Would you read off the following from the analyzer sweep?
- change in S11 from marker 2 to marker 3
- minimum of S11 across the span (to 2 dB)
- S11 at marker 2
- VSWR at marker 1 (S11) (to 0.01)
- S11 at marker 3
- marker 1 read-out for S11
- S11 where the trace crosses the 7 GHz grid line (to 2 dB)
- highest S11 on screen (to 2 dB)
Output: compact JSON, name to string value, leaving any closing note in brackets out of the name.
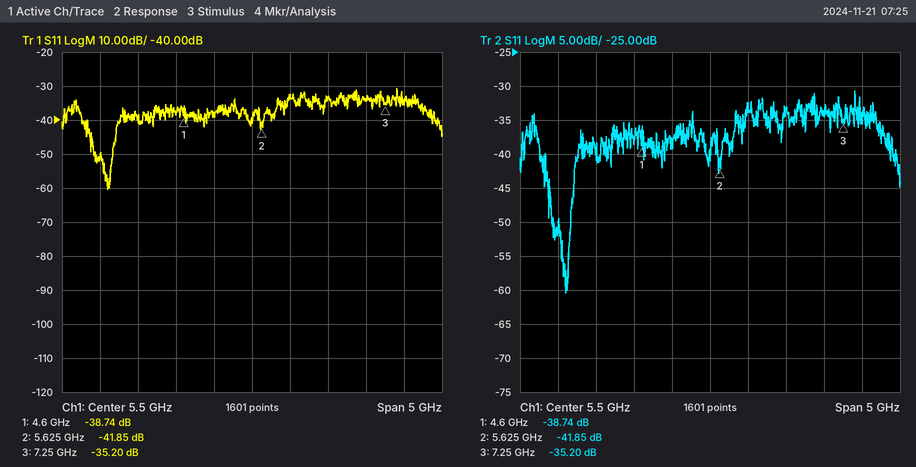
{"change in S11 from marker 2 to marker 3": "6.65 dB", "minimum of S11 across the span": "-60 dB", "S11 at marker 2": "-41.85 dB", "VSWR at marker 1 (S11)": "1.02", "S11 at marker 3": "-35.20 dB", "marker 1 read-out for S11": "-38.74 dB", "S11 where the trace crosses the 7 GHz grid line": "-34 dB", "highest S11 on screen": "-30 dB"}
